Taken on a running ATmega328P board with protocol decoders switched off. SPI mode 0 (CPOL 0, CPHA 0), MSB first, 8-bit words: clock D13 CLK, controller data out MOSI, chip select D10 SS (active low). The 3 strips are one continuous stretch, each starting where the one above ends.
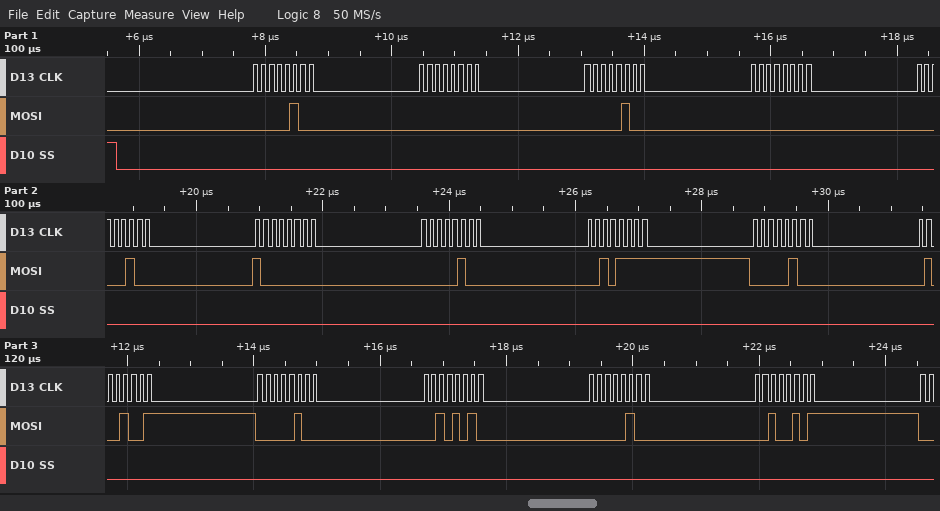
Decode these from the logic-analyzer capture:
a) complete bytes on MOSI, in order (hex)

04 00 04 00 04 80 04 2F 04 49 04 2A 04 25
